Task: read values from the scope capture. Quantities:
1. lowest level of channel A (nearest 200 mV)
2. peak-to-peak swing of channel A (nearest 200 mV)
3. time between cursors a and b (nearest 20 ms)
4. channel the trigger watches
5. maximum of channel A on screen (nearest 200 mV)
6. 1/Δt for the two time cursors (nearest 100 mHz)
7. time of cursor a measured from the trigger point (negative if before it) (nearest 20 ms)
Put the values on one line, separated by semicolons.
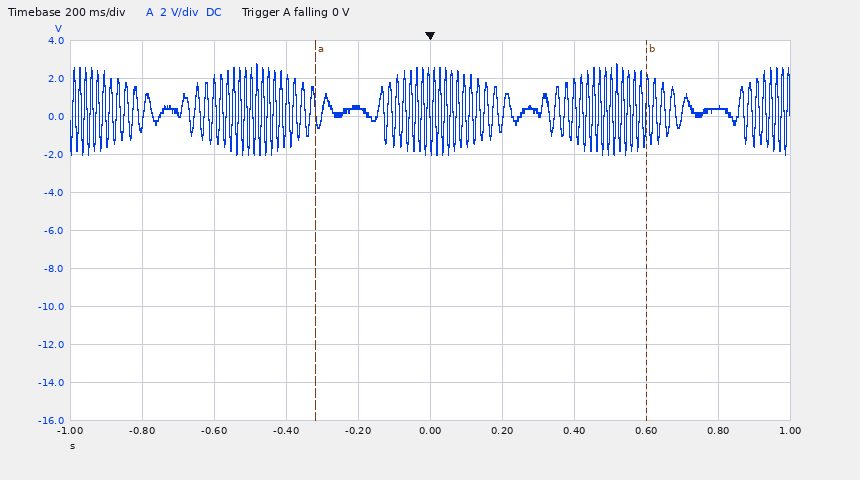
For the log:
-2.0 V; 4.8 V; 920 ms; channel A; 2.8 V; 1.1 Hz; -320 ms
